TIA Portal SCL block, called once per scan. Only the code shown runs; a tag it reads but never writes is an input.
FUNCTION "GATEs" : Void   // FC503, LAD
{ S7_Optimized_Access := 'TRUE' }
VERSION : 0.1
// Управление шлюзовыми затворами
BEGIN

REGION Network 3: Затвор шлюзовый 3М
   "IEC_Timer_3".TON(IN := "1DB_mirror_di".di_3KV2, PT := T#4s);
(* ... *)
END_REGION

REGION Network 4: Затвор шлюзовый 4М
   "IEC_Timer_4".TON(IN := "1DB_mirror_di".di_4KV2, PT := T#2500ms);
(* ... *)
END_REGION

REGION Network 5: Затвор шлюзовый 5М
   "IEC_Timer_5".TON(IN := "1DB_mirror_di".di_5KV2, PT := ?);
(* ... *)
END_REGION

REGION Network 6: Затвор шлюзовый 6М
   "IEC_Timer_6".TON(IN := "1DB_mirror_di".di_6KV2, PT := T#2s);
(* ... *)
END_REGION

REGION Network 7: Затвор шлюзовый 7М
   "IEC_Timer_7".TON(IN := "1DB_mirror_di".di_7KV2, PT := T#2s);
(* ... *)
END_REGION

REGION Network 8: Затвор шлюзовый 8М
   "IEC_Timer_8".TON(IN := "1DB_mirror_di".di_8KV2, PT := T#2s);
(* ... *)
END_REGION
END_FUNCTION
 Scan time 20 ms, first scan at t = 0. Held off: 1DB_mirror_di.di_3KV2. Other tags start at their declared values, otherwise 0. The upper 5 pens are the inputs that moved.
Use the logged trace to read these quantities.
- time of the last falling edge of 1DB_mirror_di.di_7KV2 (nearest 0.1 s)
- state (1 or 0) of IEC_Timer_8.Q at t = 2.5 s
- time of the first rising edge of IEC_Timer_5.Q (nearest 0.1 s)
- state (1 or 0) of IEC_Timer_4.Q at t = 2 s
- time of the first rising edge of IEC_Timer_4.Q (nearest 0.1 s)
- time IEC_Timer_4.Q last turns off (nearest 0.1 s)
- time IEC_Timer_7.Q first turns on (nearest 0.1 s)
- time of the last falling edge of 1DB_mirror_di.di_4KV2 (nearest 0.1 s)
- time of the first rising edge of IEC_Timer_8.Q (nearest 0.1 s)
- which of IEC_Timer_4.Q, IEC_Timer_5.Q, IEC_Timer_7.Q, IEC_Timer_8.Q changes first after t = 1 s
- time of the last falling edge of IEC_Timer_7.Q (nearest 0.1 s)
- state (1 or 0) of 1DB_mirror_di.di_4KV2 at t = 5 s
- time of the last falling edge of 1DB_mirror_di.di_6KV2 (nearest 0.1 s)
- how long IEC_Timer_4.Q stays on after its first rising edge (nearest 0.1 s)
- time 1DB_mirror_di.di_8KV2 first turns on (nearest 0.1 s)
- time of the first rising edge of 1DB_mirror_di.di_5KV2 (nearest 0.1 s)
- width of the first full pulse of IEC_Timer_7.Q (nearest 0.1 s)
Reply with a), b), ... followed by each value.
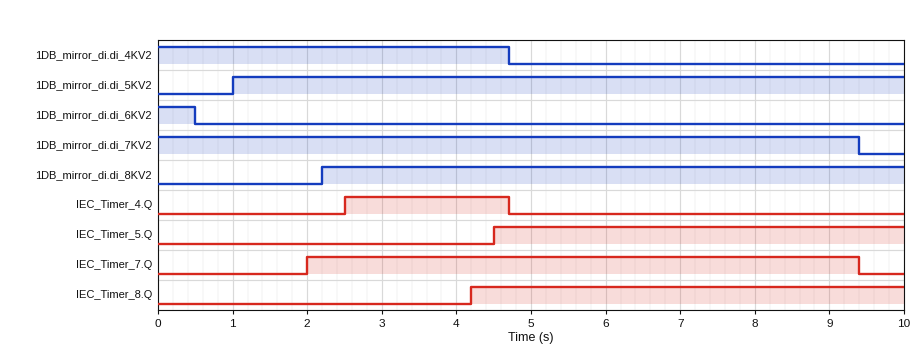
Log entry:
a) 9.4 s
b) 0
c) 4.5 s
d) 0
e) 2.5 s
f) 4.7 s
g) 2.0 s
h) 4.7 s
i) 4.2 s
j) IEC_Timer_7.Q
k) 9.4 s
l) 0
m) 0.5 s
n) 2.2 s
o) 2.2 s
p) 1.0 s
q) 7.4 s
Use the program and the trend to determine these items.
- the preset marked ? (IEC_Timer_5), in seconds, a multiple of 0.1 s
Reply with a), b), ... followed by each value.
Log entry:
a) 3.5 s
